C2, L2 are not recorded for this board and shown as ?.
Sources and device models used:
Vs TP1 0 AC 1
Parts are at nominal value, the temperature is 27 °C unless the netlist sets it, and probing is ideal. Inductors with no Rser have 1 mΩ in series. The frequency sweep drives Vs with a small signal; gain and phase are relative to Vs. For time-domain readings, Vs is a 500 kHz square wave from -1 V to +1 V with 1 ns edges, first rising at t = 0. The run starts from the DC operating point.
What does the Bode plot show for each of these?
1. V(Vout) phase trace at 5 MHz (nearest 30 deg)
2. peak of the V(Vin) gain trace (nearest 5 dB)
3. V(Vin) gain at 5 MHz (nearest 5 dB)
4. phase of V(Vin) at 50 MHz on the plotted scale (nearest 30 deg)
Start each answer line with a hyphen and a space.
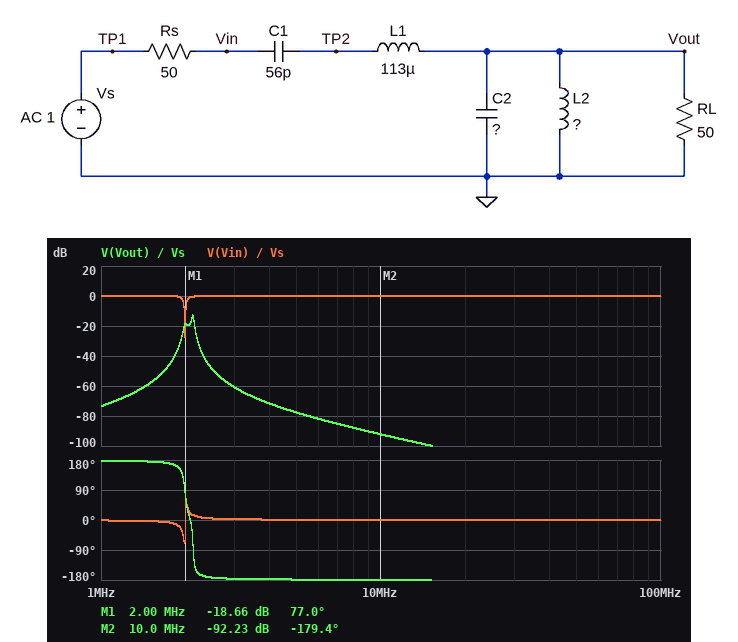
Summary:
- -180 deg
- 0 dB
- 0 dB
- 0 deg
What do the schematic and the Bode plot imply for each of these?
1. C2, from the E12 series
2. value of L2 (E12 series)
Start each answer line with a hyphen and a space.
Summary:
- 100 nF
- 56 nH
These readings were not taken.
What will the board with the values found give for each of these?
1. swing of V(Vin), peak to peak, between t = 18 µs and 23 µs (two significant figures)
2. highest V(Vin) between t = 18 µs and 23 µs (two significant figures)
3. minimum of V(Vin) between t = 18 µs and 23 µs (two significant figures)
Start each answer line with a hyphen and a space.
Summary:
- 2.1 V
- 1.0 V
- -1.0 V
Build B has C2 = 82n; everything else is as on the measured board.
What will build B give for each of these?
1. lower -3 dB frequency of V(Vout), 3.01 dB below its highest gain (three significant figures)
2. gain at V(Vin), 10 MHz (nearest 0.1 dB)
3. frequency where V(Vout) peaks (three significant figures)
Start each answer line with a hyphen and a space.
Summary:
- 2.33 MHz
- 0 dB
- 2.35 MHz
